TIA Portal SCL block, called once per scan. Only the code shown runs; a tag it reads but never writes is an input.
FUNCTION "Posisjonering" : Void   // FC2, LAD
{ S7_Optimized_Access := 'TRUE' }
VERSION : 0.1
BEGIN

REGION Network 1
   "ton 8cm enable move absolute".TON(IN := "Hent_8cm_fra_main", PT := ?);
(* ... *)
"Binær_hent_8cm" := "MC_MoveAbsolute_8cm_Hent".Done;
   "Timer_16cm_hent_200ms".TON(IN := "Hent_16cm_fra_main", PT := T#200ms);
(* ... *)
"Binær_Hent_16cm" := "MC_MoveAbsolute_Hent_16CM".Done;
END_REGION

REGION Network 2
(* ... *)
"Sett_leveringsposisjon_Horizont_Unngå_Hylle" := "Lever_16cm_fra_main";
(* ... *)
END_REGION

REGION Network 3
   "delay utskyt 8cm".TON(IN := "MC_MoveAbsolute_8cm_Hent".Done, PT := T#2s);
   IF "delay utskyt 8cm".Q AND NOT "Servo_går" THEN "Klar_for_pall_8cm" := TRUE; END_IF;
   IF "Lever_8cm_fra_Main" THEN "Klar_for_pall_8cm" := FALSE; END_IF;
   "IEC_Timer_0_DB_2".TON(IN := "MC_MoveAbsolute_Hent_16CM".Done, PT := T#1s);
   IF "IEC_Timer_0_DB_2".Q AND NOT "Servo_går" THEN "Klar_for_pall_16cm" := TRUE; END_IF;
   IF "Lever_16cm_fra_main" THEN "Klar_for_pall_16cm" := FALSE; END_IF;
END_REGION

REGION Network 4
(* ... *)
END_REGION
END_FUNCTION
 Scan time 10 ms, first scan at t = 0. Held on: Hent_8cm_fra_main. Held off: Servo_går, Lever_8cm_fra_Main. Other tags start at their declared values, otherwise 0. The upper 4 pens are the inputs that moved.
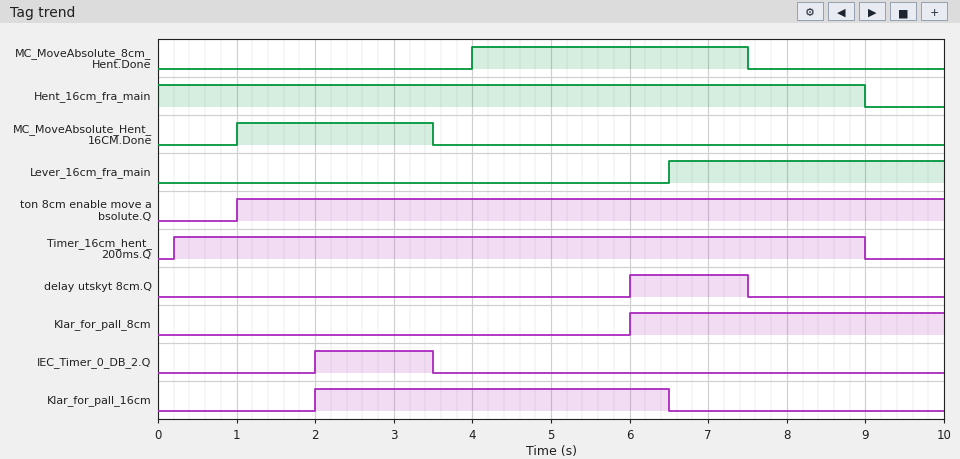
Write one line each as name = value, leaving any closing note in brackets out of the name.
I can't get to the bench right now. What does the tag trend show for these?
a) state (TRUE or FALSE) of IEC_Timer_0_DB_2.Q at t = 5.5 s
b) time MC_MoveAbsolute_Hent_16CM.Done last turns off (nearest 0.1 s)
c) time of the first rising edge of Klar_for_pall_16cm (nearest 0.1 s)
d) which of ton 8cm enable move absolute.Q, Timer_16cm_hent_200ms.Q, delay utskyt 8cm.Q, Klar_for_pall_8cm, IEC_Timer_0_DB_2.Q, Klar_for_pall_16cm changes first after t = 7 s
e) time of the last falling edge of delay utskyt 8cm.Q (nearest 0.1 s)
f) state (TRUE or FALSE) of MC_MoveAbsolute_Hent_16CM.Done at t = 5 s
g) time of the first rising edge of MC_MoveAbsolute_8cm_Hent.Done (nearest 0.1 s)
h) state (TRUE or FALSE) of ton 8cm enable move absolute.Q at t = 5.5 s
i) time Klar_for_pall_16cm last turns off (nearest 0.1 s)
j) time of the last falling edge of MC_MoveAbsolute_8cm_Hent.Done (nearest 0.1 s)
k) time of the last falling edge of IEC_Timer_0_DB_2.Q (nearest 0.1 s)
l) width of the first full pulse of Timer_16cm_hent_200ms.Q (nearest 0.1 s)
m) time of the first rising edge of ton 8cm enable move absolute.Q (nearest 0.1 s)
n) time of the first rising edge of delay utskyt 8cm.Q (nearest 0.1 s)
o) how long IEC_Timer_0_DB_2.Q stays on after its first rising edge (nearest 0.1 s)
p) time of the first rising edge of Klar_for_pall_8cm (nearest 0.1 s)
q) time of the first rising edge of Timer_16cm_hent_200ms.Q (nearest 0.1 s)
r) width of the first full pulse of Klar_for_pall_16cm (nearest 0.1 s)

state (TRUE or FALSE) of IEC_Timer_0_DB_2.Q at t = 5.5 s = FALSE
time MC_MoveAbsolute_Hent_16CM.Done last turns off = 3.5 s
time of the first rising edge of Klar_for_pall_16cm = 2.0 s
which of ton 8cm enable move absolute.Q, Timer_16cm_hent_200ms.Q, delay utskyt 8cm.Q, Klar_for_pall_8cm, IEC_Timer_0_DB_2.Q, Klar_for_pall_16cm changes first after t = 7 s = delay utskyt 8cm.Q
time of the last falling edge of delay utskyt 8cm.Q = 7.5 s
state (TRUE or FALSE) of MC_MoveAbsolute_Hent_16CM.Done at t = 5 s = FALSE
time of the first rising edge of MC_MoveAbsolute_8cm_Hent.Done = 4.0 s
state (TRUE or FALSE) of ton 8cm enable move absolute.Q at t = 5.5 s = TRUE
time Klar_for_pall_16cm last turns off = 6.5 s
time of the last falling edge of MC_MoveAbsolute_8cm_Hent.Done = 7.5 s
time of the last falling edge of IEC_Timer_0_DB_2.Q = 3.5 s
width of the first full pulse of Timer_16cm_hent_200ms.Q = 8.8 s
time of the first rising edge of ton 8cm enable move absolute.Q = 1.0 s
time of the first rising edge of delay utskyt 8cm.Q = 6.0 s
how long IEC_Timer_0_DB_2.Q stays on after its first rising edge = 1.5 s
time of the first rising edge of Klar_for_pall_8cm = 6.0 s
time of the first rising edge of Timer_16cm_hent_200ms.Q = 0.2 s
width of the first full pulse of Klar_for_pall_16cm = 4.5 s
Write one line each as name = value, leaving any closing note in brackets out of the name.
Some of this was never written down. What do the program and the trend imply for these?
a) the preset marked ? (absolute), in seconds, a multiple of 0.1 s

the preset marked ? (absolute), in seconds, a multiple of 0.1 s = 1.0 s
